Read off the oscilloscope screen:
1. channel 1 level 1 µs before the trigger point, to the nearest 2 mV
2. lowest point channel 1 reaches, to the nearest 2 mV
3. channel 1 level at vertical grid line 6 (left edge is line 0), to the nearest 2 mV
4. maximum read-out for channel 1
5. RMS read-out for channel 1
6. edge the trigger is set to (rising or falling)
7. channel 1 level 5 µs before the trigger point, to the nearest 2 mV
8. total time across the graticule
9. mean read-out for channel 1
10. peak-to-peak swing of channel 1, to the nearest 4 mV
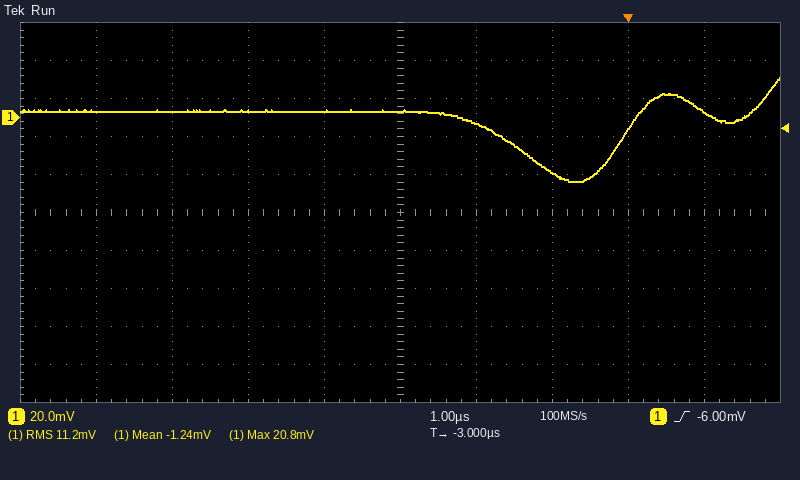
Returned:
-28 mV
-34 mV
-4 mV
20.8 mV
11.2 mV
rising
4 mV
10 µs
-1.24 mV
56 mV
